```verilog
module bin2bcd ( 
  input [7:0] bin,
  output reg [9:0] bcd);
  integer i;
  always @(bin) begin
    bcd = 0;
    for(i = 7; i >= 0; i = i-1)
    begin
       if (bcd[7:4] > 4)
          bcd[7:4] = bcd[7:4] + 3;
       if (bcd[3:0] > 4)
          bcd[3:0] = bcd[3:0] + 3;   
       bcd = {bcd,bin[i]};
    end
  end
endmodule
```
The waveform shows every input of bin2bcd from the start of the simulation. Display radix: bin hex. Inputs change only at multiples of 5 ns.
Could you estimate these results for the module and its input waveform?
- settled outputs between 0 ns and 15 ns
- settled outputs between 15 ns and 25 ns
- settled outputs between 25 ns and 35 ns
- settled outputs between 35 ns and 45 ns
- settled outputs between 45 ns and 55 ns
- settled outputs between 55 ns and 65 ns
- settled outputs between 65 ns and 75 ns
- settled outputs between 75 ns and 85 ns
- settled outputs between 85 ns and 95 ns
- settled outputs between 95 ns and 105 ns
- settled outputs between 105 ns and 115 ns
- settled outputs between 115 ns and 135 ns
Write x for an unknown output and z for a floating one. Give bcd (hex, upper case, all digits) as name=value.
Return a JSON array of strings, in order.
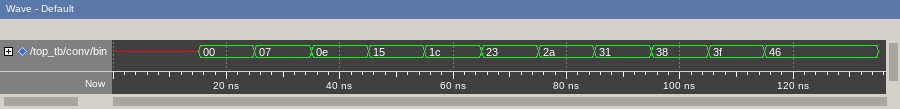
["bcd=x", "bcd=000", "bcd=007", "bcd=014", "bcd=021", "bcd=028", "bcd=035", "bcd=042", "bcd=049", "bcd=056", "bcd=063", "bcd=070"]
